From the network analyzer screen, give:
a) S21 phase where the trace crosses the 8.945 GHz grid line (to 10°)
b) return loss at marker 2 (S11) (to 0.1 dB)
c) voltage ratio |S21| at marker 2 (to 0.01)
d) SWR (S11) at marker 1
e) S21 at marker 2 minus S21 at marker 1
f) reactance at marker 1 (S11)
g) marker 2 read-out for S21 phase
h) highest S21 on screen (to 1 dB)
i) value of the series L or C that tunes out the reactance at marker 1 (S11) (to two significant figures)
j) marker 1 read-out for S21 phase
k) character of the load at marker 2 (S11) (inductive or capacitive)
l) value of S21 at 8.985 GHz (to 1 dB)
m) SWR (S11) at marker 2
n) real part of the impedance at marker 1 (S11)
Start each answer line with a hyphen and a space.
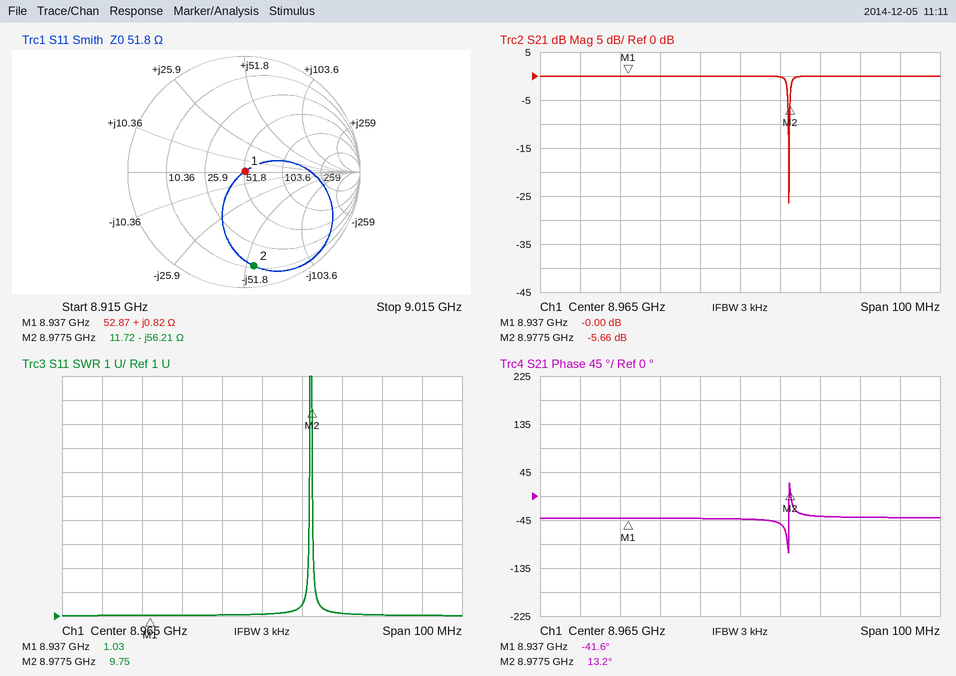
- -40°
- 1.8 dB
- 0.52
- 1.03
- -5.66 dB
- +0.82 Ω
- 13.2°
- 0 dB
- 22 pF
- -41.6°
- capacitive
- 0 dB
- 9.75
- 52.87 Ω
